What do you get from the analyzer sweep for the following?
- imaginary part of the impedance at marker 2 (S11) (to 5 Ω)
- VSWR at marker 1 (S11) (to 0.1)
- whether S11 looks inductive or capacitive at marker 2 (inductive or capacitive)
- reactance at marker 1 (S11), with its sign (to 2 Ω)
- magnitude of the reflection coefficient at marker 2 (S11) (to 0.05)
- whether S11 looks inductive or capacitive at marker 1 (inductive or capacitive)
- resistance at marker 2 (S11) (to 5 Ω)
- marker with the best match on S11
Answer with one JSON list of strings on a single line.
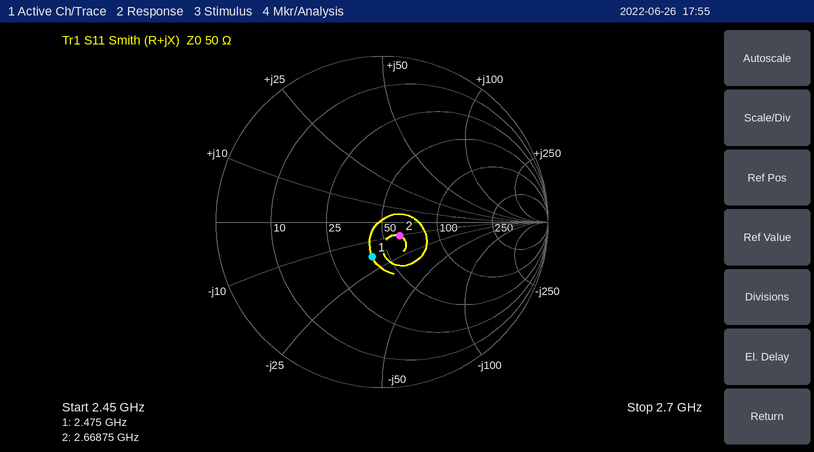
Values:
["-10 Ω", "1.6", "capacitive", "-18 Ω", "0.15", "capacitive", "60 Ω", "marker 2"]
